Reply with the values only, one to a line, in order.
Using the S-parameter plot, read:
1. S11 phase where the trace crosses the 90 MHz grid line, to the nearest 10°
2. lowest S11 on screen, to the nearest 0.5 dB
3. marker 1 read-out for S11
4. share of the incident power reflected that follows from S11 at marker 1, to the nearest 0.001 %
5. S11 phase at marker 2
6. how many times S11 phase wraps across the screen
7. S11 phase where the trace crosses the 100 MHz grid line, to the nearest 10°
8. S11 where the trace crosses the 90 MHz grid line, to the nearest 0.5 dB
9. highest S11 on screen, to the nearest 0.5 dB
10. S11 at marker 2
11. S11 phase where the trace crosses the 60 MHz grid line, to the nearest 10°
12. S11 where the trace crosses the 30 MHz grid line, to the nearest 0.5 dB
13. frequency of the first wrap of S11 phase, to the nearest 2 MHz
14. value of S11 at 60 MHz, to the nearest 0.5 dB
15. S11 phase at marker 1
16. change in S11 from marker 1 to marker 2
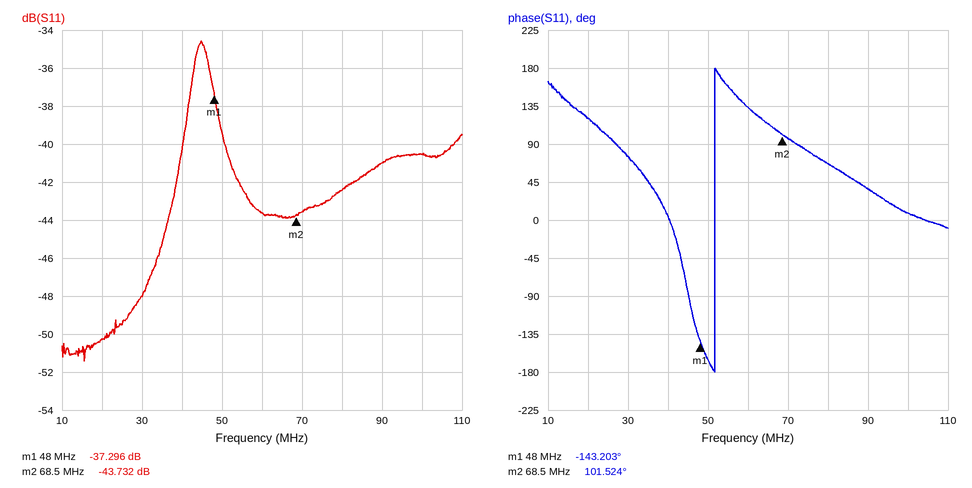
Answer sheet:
40°
-51.5 dB
-37.296 dB
0.019 %
101.524°
1
10°
-41.0 dB
-34.5 dB
-43.732 dB
130°
-48.0 dB
52 MHz
-43.5 dB
-143.203°
-6.436 dB
